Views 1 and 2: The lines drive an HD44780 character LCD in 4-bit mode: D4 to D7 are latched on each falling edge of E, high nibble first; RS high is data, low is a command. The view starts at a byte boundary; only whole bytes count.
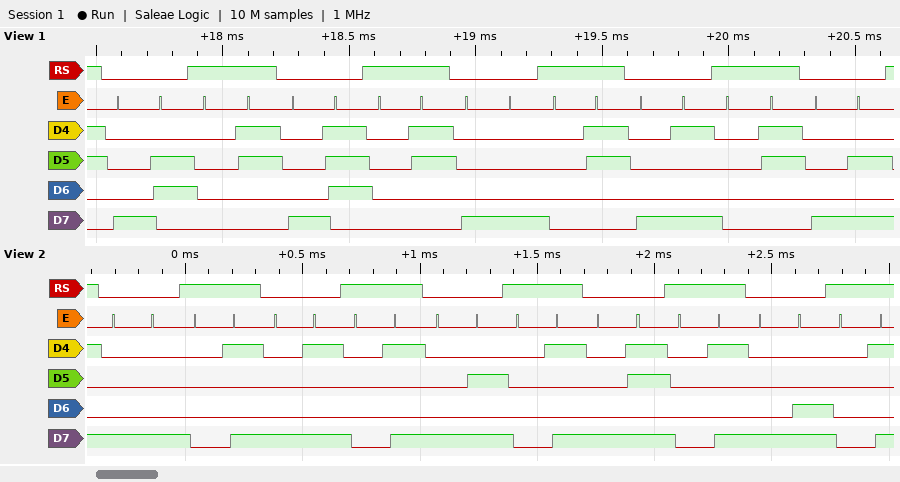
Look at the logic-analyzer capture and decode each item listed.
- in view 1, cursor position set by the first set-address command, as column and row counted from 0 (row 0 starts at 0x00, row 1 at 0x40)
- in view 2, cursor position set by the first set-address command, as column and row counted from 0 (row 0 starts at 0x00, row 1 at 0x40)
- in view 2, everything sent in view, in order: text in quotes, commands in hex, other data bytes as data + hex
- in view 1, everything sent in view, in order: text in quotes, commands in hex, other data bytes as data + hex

column 6, row 0
column 8, row 0
0x88 data 09 0x89 data 09 0x8A data 09 0x8B data 09 0x8C data 09
0x86 data 03 0x87 data 03 0x88 data 03 0x89 data 03 0x8A
